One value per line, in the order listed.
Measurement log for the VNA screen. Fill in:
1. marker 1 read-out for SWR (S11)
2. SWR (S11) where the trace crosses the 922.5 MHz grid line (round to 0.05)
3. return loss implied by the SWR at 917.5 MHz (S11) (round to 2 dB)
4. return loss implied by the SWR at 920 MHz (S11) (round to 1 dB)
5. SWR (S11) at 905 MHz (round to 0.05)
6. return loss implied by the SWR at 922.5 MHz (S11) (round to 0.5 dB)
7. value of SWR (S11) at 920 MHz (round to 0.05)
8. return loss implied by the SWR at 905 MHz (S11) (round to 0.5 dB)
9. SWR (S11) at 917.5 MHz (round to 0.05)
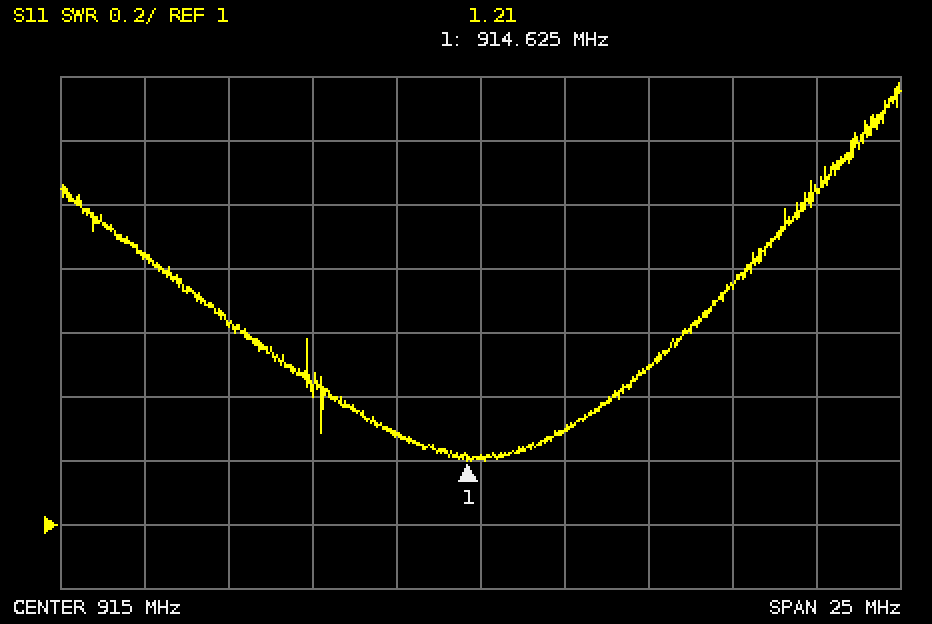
1.21
1.75
18 dB
14 dB
1.85
11.5 dB
1.50
10.5 dB
1.30
